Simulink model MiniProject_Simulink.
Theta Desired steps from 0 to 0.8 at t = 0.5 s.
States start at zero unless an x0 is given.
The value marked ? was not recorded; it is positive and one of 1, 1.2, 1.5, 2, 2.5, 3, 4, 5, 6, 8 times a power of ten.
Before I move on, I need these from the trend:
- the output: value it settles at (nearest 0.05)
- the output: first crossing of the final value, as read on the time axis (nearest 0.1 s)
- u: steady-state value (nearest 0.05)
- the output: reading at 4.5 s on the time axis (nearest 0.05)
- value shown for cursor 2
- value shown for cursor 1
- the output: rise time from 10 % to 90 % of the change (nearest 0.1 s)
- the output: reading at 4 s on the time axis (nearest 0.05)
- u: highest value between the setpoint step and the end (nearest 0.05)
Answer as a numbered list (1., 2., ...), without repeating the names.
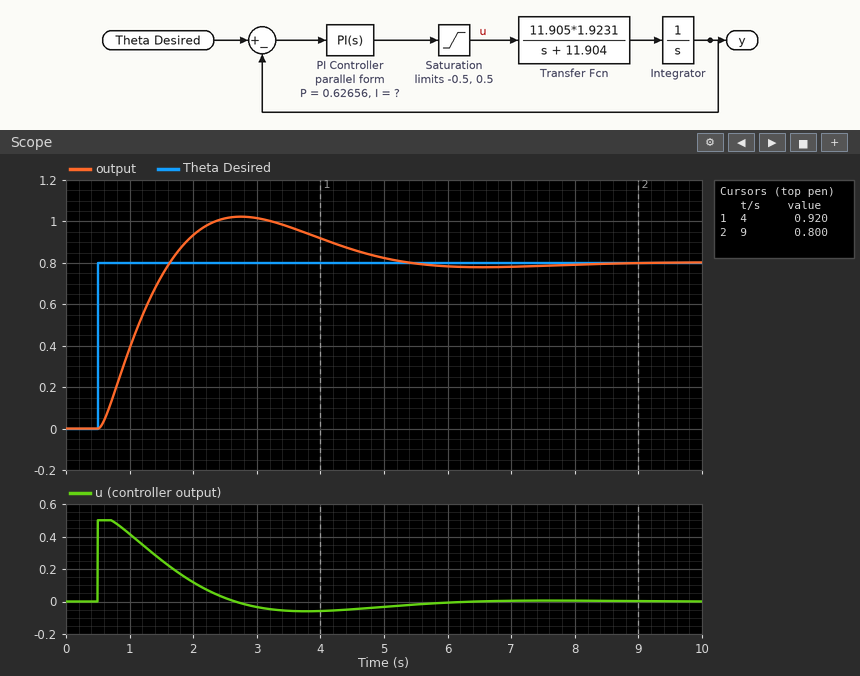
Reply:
1. 0.80
2. 1.6 s
3. 0.00
4. 0.85
5. 0.800
6. 0.920
7. 0.8 s
8. 0.90
9. 0.50
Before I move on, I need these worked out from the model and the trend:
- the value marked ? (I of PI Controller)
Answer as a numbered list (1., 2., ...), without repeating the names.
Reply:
1. 0.5
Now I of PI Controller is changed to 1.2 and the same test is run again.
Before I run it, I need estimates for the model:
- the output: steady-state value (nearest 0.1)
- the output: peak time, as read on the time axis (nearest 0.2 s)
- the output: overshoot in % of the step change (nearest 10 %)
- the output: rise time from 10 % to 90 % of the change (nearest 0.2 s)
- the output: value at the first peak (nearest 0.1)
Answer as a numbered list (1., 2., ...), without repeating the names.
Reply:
1. 0.8
2. 2.2 s
3. 50 %
4. 0.6 s
5. 1.2
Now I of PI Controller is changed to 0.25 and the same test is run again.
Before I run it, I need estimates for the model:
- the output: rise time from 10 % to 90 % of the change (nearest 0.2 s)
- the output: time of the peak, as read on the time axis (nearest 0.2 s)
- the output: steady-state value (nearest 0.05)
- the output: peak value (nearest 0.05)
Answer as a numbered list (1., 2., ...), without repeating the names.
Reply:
1. 1.0 s
2. 3.4 s
3. 0.80
4. 0.95
